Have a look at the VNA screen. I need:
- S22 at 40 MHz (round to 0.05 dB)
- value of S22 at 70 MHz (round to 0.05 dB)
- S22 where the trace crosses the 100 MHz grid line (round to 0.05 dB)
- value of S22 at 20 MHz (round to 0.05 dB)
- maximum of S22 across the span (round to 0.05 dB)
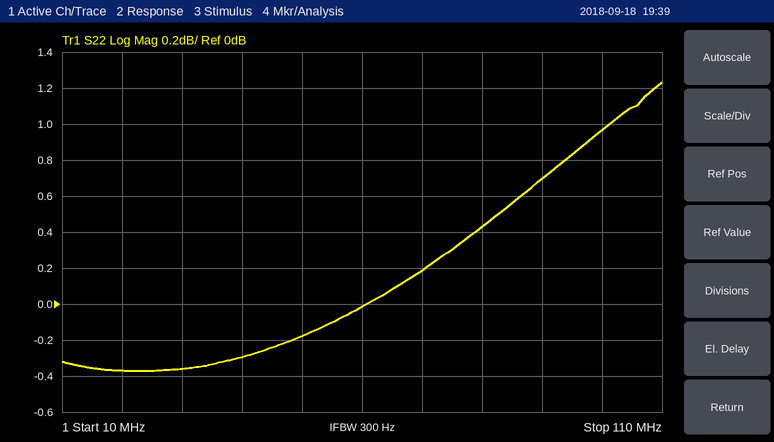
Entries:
-0.30 dB
0.20 dB
0.95 dB
-0.35 dB
1.25 dB
